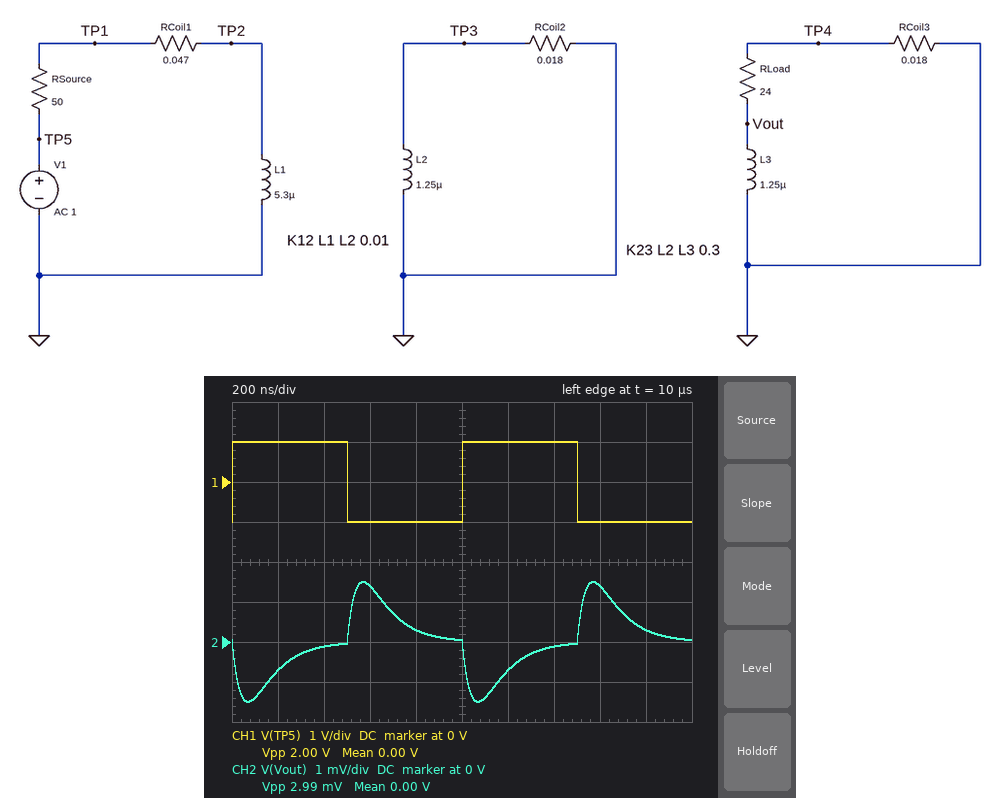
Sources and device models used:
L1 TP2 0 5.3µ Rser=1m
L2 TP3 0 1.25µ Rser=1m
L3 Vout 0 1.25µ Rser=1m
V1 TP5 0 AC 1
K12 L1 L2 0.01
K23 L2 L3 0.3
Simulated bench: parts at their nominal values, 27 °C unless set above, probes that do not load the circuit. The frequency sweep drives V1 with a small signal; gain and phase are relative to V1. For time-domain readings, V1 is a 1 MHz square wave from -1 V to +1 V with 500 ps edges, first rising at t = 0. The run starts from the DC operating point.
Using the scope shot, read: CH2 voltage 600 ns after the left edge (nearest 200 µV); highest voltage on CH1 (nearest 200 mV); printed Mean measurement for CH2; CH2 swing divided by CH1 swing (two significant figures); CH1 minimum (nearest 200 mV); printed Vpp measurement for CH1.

1.4 mV
1.0 V
0.00 V
0.0015
-1.0 V
2.00 V
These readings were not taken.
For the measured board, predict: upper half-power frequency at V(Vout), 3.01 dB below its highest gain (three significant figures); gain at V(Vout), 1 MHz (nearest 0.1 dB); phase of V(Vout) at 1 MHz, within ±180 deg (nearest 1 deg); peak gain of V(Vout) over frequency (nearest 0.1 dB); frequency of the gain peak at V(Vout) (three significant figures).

5.74 MHz
-62.2 dB
-140 deg
-59.9 dB
2.25 MHz
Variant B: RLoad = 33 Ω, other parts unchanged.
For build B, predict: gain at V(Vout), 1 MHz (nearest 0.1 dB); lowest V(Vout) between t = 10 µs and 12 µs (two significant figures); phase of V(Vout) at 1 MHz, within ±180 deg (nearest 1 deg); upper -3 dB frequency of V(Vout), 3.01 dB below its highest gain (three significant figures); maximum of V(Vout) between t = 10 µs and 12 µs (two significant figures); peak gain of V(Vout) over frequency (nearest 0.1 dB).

-62.1 dB
-1.7 mV
-136 deg
7.10 MHz
1.7 mV
-59.2 dB
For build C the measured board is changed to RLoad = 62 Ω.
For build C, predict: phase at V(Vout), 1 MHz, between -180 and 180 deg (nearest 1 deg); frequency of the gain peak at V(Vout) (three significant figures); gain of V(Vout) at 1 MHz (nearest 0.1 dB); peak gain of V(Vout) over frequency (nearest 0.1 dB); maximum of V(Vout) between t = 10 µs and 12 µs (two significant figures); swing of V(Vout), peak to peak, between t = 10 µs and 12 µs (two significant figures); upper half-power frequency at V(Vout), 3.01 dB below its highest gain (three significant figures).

-130 deg
3.61 MHz
-61.9 dB
-58.1 dB
2.0 mV
4.0 mV
11.3 MHz
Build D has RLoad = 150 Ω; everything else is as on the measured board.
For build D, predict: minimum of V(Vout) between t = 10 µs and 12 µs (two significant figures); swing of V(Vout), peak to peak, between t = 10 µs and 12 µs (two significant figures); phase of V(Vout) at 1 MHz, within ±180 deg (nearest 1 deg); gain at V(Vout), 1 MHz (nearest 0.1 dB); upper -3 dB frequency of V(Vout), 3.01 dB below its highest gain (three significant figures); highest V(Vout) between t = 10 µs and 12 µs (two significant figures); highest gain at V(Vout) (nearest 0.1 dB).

-2.4 mV
4.7 mV
-126 deg
-61.9 dB
23.8 MHz
2.4 mV
-57.3 dB
